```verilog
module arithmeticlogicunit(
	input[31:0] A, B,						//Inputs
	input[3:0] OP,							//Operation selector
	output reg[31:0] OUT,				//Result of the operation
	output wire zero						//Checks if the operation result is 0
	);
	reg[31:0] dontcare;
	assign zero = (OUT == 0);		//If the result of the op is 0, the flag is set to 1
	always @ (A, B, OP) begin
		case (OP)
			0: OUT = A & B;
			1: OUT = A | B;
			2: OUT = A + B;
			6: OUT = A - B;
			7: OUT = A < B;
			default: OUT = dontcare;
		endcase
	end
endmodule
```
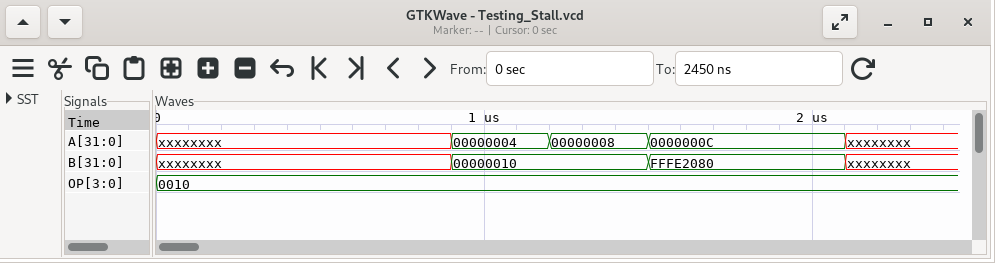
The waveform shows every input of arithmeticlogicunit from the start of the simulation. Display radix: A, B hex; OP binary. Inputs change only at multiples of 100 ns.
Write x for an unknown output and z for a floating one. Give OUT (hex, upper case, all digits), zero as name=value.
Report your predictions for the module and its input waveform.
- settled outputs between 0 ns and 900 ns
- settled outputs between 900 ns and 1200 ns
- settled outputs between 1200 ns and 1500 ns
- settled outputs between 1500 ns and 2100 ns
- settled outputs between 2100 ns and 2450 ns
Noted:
OUT=x, zero=x
OUT=00000014, zero=0
OUT=00000018, zero=0
OUT=FFFE208C, zero=0
OUT=x, zero=x
